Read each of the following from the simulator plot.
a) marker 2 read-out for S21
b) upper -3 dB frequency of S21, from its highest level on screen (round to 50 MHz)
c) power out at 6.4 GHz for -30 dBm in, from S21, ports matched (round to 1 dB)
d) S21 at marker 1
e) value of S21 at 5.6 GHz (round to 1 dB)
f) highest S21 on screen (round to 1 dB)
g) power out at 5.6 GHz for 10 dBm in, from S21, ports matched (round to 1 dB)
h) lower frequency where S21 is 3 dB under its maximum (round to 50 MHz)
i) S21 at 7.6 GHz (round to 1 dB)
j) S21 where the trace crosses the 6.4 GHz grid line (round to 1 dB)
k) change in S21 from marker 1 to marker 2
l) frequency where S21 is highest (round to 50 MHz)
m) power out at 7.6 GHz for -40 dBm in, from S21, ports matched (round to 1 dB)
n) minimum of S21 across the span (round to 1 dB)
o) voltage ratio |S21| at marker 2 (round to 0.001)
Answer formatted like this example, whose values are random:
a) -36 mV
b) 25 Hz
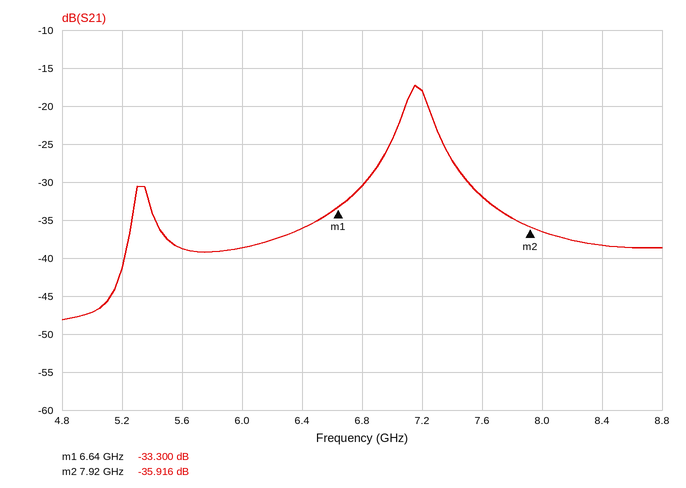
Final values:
a) -35.916 dB
b) 7.25 GHz
c) -66 dBm
d) -33.300 dB
e) -39 dB
f) -17 dB
g) -29 dBm
h) 7.10 GHz
i) -32 dB
j) -36 dB
k) -2.616 dB
l) 7.15 GHz
m) -72 dBm
n) -48 dB
o) 0.016
